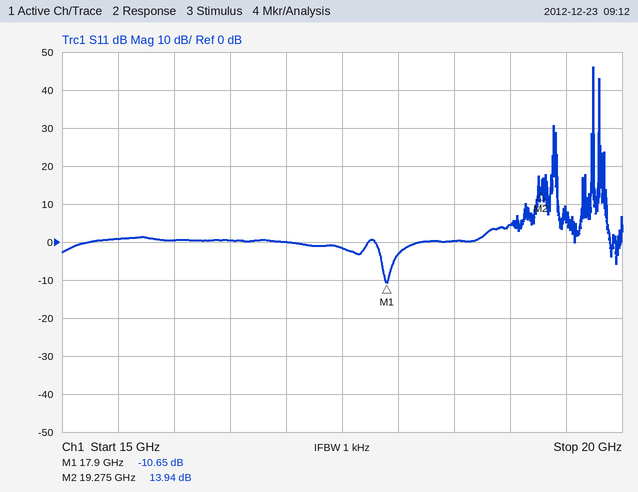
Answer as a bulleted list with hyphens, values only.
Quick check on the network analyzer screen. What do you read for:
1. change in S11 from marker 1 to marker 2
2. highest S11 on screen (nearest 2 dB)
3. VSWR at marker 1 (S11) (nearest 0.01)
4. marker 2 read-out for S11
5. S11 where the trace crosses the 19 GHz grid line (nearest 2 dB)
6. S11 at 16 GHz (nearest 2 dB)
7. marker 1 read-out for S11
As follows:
- 24.59 dB
- 46 dB
- 1.83
- 13.94 dB
- 4 dB
- 0 dB
- -10.65 dB
